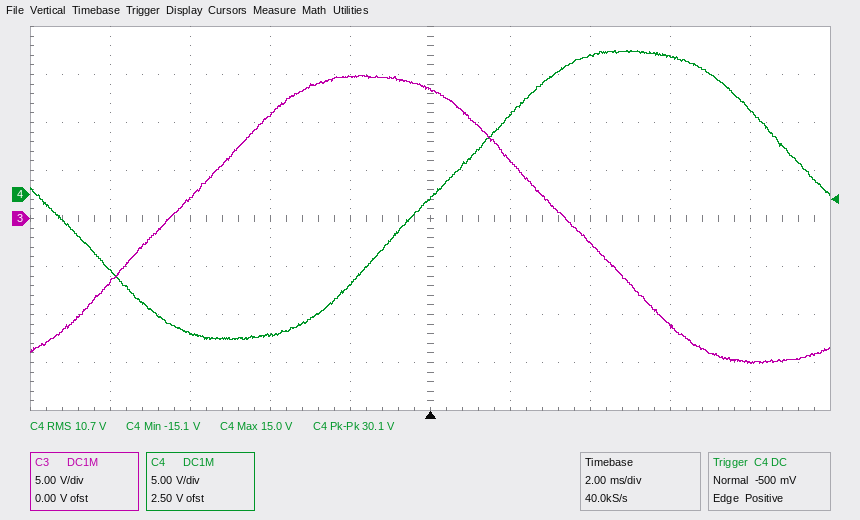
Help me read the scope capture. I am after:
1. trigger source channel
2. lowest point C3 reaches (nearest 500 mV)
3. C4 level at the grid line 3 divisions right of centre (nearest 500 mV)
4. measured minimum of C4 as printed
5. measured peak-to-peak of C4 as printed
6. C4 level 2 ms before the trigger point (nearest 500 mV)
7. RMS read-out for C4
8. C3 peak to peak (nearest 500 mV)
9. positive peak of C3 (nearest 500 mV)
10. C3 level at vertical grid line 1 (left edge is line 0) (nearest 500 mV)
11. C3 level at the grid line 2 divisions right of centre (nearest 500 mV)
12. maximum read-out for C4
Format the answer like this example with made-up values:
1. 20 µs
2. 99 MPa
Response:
1. C4
2. -15.0 V
3. 14.5 V
4. -15.1 V
5. 30.1 V
6. -9.5 V
7. 10.7 V
8. 30.0 V
9. 15.0 V
10. -6.5 V
11. -2.5 V
12. 15.0 V
